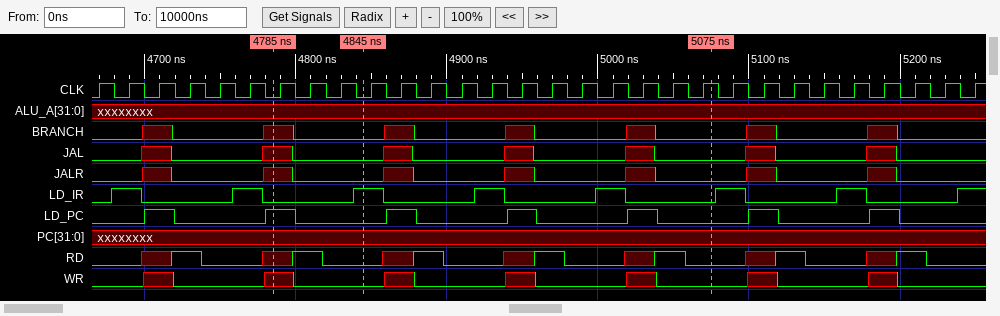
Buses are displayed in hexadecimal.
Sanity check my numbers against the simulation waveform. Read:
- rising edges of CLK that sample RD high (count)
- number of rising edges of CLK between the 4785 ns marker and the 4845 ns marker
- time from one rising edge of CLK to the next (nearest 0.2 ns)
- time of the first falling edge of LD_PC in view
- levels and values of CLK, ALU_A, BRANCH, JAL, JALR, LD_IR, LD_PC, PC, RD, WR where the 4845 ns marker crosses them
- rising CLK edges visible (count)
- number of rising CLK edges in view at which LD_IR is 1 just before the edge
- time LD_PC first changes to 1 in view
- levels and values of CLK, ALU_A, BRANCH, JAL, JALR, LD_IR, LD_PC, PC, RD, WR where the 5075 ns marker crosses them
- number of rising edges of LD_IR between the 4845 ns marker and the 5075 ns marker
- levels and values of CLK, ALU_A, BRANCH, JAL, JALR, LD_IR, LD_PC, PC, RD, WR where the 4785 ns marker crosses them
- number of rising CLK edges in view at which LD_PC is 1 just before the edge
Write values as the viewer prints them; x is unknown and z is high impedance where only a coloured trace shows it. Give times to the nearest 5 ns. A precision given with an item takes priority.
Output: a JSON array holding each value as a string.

["7", "3", "20 ns", "4720 ns", "CLK=0, ALU_A=xxxxxxxx, BRANCH=0, JAL=0, JALR=0, LD_IR=1, LD_PC=0, PC=xxxxxxxx, RD=0, WR=0", "30", "8", "4700 ns", "CLK=1, ALU_A=xxxxxxxx, BRANCH=0, JAL=0, JALR=0, LD_IR=0, LD_PC=0, PC=xxxxxxxx, RD=0, WR=0", "2", "CLK=0, ALU_A=xxxxxxxx, BRANCH=x, JAL=x, JALR=x, LD_IR=0, LD_PC=1, PC=xxxxxxxx, RD=x, WR=x", "7"]
